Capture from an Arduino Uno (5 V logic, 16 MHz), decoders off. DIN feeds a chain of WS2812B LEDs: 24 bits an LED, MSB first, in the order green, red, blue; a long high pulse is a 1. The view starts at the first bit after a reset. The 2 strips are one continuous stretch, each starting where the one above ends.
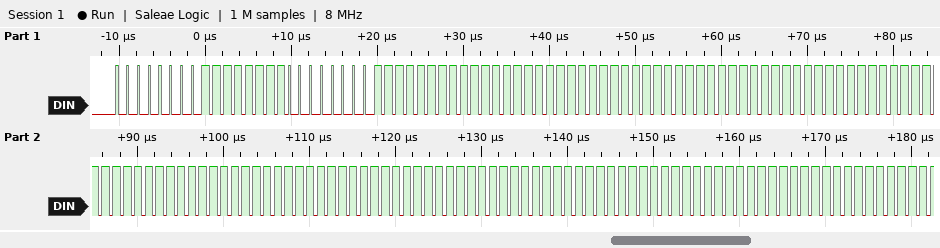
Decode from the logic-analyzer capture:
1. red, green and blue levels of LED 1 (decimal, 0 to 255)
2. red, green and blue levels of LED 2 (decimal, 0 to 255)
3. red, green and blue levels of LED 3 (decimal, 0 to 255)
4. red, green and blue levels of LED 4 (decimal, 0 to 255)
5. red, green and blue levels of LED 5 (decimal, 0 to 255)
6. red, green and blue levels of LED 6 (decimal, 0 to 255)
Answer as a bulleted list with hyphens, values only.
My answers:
- 255, 0, 0
- 255, 255, 255
- 255, 255, 255
- 255, 255, 255
- 255, 255, 255
- 255, 255, 255
